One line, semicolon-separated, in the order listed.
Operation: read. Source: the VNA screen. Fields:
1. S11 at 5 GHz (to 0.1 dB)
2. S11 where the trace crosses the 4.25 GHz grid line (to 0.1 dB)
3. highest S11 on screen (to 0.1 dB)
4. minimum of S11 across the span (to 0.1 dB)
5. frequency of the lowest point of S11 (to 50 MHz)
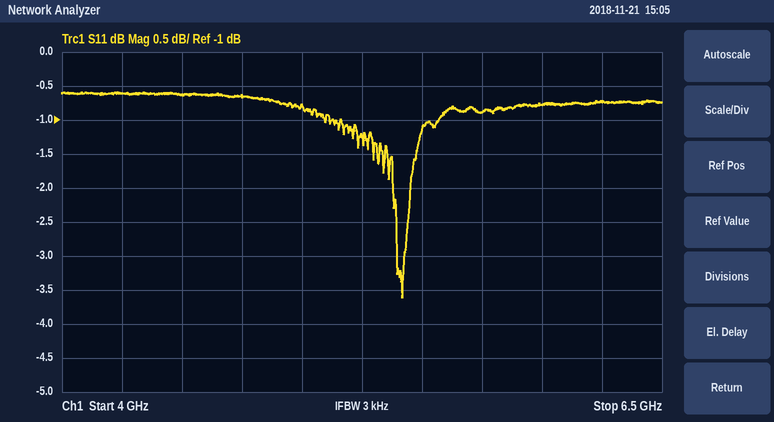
-0.8 dB; -0.6 dB; -0.6 dB; -3.6 dB; 5.40 GHz
